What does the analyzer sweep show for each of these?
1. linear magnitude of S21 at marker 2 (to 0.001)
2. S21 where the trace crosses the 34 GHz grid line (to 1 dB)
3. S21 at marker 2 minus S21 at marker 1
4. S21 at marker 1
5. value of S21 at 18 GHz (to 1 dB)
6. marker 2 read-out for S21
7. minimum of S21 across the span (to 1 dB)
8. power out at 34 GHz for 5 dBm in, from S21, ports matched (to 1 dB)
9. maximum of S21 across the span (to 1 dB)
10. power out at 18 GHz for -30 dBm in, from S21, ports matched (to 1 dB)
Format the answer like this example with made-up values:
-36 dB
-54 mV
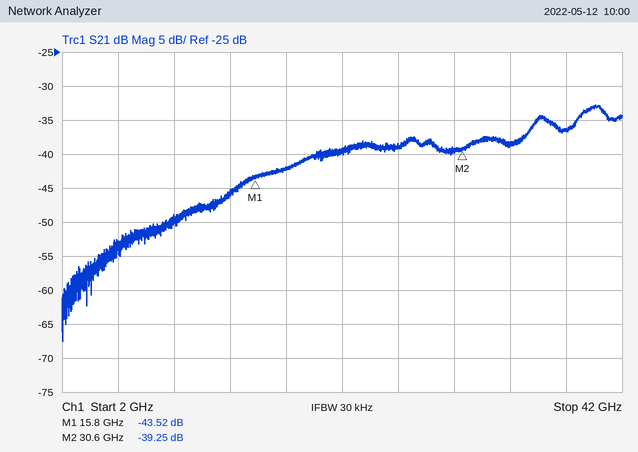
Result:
0.011
-39 dB
4.27 dB
-43.52 dB
-42 dB
-39.25 dB
-68 dB
-34 dBm
-33 dB
-72 dBm
